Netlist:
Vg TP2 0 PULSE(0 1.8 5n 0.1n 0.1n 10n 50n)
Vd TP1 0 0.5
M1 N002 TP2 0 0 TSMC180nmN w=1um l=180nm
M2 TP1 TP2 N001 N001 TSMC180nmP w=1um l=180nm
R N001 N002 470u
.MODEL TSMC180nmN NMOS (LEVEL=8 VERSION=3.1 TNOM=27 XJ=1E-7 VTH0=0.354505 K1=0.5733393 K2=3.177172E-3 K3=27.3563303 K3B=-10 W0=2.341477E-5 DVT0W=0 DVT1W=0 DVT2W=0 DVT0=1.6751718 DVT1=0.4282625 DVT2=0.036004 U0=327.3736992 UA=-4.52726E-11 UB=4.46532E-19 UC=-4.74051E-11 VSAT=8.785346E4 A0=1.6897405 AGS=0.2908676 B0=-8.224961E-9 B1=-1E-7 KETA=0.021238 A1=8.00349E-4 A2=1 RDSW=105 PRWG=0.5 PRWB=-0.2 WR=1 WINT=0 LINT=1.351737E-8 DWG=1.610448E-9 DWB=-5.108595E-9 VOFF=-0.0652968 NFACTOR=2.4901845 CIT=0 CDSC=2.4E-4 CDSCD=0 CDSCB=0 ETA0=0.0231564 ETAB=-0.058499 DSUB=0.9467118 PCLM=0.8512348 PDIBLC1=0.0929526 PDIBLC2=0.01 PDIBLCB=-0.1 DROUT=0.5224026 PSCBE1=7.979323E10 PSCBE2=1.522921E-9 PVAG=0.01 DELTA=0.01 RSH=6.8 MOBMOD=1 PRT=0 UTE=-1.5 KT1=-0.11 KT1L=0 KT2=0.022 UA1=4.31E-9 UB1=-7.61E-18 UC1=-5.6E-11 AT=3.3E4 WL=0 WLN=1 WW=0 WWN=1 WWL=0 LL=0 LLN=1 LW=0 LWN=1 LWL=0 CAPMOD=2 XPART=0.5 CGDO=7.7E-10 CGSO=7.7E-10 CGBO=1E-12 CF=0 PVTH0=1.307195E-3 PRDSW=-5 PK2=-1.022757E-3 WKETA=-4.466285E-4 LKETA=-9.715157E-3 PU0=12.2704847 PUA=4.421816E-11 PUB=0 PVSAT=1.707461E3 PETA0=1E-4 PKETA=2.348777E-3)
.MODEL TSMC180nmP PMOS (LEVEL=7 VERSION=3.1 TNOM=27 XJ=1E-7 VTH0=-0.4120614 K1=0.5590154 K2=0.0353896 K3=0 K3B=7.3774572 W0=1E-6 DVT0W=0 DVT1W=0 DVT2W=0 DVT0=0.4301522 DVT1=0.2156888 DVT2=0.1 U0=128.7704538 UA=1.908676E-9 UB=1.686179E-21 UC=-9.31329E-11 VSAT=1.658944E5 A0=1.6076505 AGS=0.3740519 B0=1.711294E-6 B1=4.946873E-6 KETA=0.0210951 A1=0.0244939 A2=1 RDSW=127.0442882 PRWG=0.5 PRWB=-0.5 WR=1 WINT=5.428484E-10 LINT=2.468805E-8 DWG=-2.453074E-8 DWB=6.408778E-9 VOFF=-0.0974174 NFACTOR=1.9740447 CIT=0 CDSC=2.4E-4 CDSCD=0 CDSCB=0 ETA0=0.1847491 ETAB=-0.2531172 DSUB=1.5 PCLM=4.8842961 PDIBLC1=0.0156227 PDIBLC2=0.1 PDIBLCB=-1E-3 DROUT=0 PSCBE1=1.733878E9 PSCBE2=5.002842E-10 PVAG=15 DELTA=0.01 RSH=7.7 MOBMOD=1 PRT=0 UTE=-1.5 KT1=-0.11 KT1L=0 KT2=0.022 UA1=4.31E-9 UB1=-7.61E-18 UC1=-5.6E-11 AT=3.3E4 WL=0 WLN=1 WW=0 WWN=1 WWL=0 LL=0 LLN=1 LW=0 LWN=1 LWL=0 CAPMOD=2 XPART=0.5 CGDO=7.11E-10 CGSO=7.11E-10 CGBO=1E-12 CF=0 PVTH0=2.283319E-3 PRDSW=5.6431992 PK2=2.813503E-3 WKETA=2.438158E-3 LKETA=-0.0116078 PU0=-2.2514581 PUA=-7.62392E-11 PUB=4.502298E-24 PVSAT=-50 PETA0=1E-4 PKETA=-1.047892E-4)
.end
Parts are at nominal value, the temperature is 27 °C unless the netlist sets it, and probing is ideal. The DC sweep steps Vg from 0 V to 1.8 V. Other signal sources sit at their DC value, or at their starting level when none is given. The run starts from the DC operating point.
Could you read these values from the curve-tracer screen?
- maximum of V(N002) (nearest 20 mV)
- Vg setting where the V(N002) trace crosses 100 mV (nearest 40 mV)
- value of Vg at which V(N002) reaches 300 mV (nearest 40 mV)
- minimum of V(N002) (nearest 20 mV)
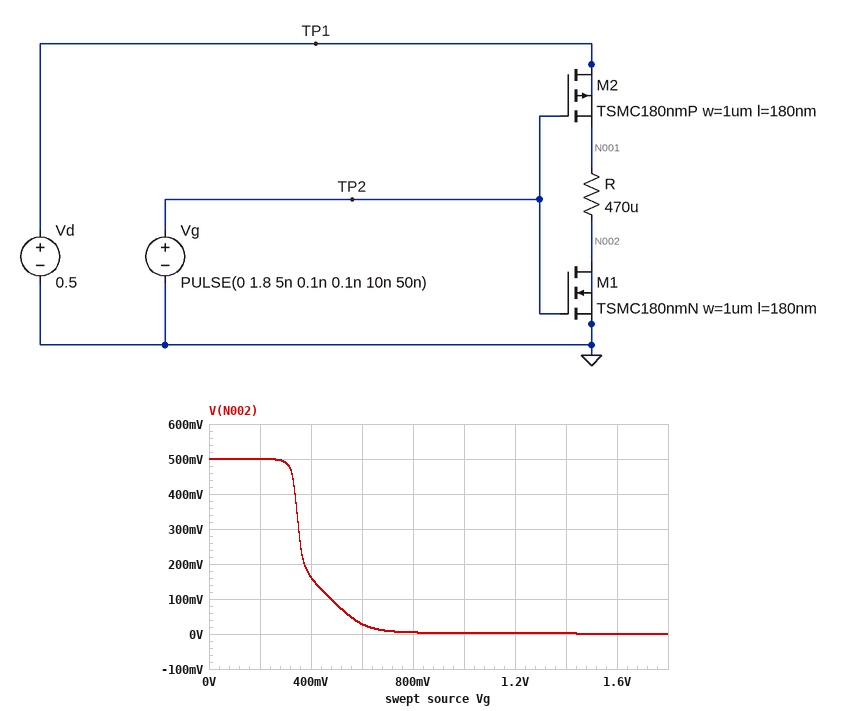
500 mV
480 mV
360 mV
0 V
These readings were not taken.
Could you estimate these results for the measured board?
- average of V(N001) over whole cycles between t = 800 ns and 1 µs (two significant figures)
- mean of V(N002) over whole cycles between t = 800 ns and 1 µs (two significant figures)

390 mV
390 mV
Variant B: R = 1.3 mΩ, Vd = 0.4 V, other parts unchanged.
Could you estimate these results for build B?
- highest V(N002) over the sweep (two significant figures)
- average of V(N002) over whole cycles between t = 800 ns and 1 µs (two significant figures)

400 mV
270 mV
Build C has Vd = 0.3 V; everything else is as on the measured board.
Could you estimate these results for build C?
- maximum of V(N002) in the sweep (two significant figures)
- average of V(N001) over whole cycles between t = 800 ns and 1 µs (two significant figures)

300 mV
67 mV
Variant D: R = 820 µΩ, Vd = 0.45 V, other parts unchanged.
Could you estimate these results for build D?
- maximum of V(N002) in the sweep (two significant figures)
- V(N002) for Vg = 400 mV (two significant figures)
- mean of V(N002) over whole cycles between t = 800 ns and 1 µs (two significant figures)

450 mV
110 mV
330 mV
